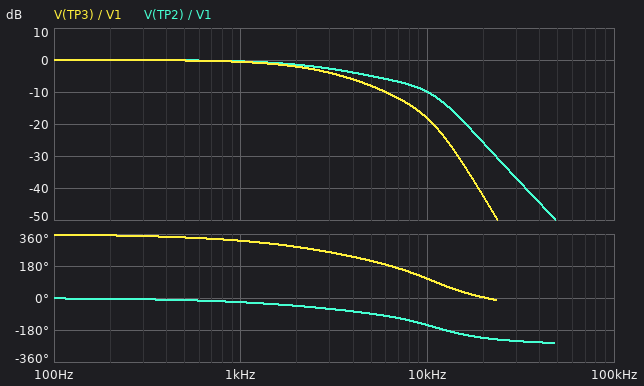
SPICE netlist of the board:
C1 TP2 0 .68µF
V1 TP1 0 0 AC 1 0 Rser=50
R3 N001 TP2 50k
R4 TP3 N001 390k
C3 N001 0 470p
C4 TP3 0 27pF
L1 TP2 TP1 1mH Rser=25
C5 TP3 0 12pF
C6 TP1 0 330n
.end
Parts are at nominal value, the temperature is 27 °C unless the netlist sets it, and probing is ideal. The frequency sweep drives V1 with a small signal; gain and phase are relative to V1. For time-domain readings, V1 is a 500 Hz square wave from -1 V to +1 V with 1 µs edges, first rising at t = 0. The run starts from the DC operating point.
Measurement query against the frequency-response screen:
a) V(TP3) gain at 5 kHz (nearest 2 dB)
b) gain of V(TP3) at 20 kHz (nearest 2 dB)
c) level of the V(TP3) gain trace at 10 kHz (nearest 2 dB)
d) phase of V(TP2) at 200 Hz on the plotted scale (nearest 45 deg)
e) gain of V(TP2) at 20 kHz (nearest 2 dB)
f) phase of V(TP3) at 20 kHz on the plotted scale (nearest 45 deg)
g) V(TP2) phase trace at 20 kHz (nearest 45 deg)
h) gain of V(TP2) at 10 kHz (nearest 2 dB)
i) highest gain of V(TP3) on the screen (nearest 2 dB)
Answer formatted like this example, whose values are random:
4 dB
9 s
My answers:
-8 dB
-42 dB
-18 dB
0 deg
-26 dB
0 deg
-225 deg
-10 dB
0 dB
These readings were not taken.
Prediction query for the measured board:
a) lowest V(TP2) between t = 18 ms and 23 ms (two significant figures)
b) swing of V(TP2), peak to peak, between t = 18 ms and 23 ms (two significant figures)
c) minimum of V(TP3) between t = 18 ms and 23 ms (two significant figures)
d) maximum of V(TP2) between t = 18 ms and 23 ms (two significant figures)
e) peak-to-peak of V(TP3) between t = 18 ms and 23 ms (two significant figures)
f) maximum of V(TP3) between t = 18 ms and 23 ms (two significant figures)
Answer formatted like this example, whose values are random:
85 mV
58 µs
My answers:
-1.0 V
2.0 V
-1.0 V
1.0 V
2.0 V
1.0 V
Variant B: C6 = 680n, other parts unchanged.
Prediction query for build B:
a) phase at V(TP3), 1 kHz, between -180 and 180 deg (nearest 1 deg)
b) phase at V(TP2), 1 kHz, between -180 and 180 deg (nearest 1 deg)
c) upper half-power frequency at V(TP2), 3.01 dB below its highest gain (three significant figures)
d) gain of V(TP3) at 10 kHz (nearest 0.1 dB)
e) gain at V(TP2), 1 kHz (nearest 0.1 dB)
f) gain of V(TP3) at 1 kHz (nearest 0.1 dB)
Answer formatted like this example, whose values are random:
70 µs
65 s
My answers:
-44 deg
-29 deg
2.46 kHz
-20.3 dB
-0.7 dB
-0.9 dB
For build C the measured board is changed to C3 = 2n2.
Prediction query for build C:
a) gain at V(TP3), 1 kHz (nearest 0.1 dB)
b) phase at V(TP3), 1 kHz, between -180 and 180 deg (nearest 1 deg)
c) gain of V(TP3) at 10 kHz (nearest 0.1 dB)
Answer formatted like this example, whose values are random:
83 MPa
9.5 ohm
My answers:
-2.2 dB
-64 deg
-29.8 dB
